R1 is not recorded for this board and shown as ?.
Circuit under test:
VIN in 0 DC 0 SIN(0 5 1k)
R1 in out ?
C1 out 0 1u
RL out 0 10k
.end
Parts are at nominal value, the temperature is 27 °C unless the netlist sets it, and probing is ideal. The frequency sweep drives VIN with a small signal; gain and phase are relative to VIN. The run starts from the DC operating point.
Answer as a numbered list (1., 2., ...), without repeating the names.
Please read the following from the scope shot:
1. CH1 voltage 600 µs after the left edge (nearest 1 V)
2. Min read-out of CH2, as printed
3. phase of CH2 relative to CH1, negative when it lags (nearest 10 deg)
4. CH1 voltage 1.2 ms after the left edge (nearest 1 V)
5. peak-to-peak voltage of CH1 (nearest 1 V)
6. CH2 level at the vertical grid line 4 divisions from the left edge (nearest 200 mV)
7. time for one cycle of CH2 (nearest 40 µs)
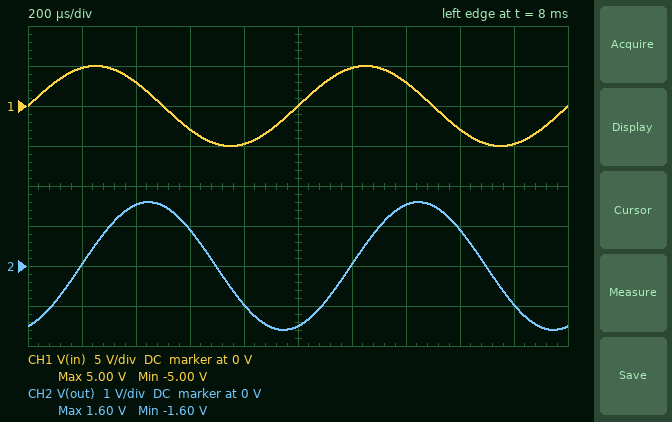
1. -3 V
2. -1.60 V
3. -70 deg
4. 5 V
5. 10 V
6. -1.0 V
7. 1.00 ms
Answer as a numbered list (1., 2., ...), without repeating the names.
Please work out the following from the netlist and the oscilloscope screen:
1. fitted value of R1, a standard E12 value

1. 470 Ω
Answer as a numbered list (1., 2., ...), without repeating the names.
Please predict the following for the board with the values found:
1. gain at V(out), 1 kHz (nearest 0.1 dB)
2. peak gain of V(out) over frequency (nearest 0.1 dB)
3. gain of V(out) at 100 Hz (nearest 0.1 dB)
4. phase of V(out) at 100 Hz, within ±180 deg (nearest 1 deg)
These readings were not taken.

1. -9.9 dB
2. -0.4 dB
3. -0.7 dB
4. -16 deg
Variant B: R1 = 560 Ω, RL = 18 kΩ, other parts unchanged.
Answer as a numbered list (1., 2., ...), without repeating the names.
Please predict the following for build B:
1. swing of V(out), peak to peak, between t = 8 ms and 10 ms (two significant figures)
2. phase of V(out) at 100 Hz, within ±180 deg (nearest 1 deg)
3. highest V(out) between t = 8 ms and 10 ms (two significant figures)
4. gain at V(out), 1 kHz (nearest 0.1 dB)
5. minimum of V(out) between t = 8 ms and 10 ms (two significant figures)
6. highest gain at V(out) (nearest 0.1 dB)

1. 2.7 V
2. -19 deg
3. 1.4 V
4. -11.3 dB
5. -1.4 V
6. -0.3 dB
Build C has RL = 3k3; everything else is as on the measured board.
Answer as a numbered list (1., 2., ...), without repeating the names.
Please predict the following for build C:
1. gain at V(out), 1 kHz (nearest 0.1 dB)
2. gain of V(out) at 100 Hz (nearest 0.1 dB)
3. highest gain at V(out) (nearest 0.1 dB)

1. -10.0 dB
2. -1.4 dB
3. -1.2 dB
